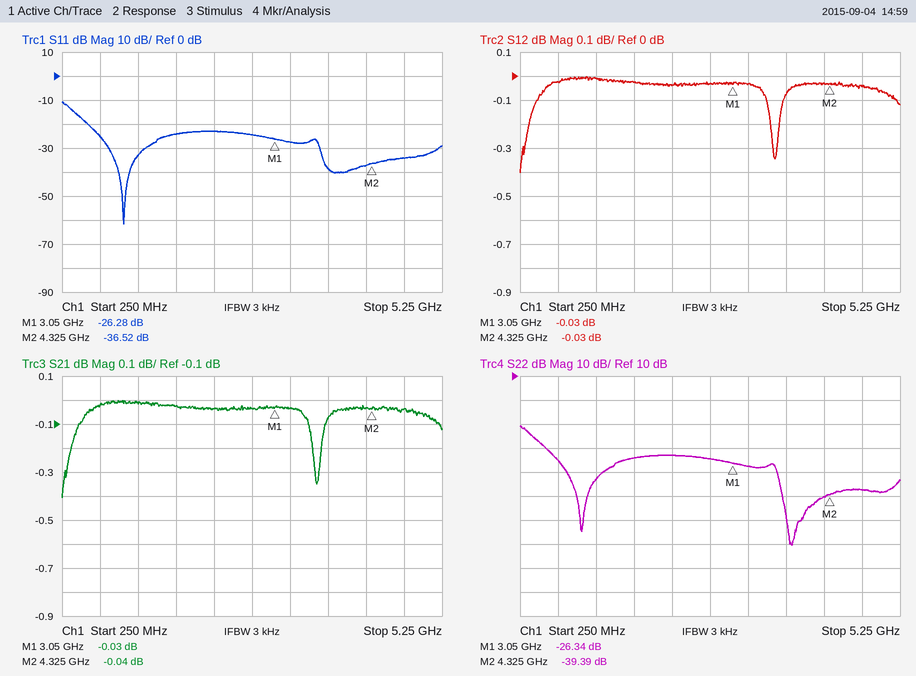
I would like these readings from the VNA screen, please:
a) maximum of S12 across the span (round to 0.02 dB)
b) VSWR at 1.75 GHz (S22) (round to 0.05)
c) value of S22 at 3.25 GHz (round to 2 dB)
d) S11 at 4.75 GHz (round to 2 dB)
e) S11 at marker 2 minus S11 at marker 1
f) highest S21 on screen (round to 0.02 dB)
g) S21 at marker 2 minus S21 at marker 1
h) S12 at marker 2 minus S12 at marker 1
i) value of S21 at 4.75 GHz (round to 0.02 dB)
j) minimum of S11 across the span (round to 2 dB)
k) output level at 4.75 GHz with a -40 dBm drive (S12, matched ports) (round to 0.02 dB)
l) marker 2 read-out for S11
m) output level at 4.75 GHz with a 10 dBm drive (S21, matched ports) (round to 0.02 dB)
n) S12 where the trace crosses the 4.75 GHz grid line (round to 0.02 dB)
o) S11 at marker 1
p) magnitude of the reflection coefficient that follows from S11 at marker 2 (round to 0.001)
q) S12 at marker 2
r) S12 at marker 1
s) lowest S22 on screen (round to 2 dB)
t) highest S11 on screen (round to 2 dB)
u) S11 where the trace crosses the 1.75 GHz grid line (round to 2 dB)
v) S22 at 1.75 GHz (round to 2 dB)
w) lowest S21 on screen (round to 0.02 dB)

0.00 dB
1.15
-28 dB
-34 dB
-10.24 dB
0.00 dB
-0.01 dB
0.00 dB
-0.04 dB
-62 dB
-40.04 dBm
-36.52 dB
9.96 dBm
-0.04 dB
-26.28 dB
0.015
-0.03 dB
-0.03 dB
-60 dB
-10 dB
-24 dB
-24 dB
-0.40 dB
